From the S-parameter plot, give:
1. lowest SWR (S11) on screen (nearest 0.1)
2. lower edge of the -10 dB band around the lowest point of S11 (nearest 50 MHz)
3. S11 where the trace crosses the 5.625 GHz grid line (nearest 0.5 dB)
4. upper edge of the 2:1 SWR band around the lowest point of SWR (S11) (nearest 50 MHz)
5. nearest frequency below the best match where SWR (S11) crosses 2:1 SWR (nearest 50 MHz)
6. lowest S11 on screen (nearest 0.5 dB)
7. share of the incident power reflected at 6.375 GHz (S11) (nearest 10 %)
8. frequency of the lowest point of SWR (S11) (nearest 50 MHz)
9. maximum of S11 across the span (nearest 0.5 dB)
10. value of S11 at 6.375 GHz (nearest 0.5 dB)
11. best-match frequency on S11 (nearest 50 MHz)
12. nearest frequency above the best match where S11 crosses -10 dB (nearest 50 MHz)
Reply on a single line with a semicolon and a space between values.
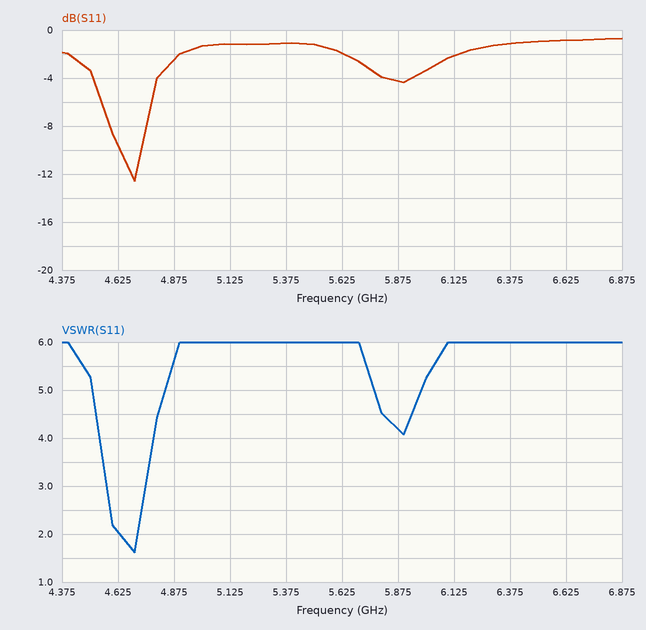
1.6; 4.65 GHz; -2.0 dB; 4.70 GHz; 4.65 GHz; -12.5 dB; 80 %; 4.70 GHz; -0.5 dB; -1.0 dB; 4.70 GHz; 4.75 GHz
